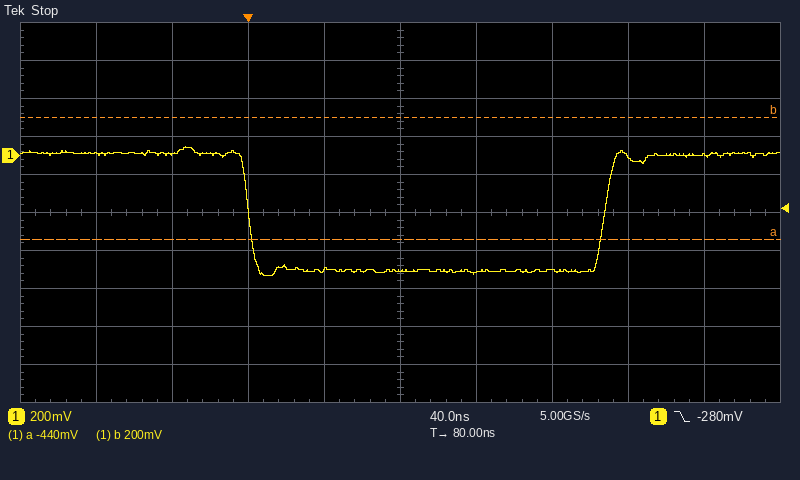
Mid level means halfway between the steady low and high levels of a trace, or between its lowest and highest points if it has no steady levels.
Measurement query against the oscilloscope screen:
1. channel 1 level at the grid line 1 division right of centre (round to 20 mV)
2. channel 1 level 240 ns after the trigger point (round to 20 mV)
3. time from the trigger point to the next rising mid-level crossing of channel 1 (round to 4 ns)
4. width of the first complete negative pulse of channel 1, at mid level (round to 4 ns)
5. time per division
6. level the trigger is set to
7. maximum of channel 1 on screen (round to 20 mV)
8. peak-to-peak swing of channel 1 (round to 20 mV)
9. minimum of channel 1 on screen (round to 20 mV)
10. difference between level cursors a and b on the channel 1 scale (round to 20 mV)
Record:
-620 mV
0 mV
188 ns
188 ns
40 ns
-280 mV
40 mV
680 mV
-640 mV
640 mV
